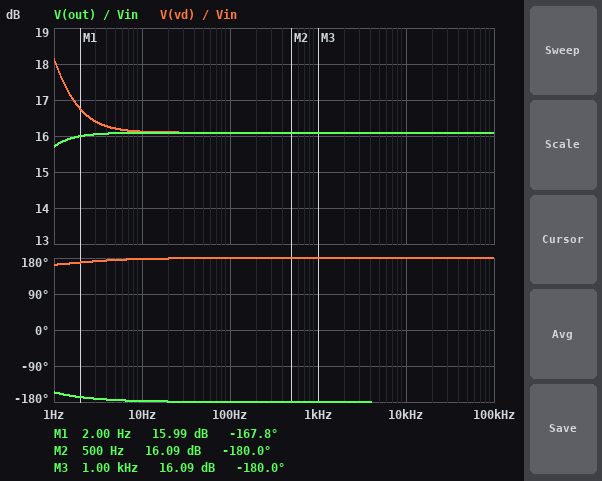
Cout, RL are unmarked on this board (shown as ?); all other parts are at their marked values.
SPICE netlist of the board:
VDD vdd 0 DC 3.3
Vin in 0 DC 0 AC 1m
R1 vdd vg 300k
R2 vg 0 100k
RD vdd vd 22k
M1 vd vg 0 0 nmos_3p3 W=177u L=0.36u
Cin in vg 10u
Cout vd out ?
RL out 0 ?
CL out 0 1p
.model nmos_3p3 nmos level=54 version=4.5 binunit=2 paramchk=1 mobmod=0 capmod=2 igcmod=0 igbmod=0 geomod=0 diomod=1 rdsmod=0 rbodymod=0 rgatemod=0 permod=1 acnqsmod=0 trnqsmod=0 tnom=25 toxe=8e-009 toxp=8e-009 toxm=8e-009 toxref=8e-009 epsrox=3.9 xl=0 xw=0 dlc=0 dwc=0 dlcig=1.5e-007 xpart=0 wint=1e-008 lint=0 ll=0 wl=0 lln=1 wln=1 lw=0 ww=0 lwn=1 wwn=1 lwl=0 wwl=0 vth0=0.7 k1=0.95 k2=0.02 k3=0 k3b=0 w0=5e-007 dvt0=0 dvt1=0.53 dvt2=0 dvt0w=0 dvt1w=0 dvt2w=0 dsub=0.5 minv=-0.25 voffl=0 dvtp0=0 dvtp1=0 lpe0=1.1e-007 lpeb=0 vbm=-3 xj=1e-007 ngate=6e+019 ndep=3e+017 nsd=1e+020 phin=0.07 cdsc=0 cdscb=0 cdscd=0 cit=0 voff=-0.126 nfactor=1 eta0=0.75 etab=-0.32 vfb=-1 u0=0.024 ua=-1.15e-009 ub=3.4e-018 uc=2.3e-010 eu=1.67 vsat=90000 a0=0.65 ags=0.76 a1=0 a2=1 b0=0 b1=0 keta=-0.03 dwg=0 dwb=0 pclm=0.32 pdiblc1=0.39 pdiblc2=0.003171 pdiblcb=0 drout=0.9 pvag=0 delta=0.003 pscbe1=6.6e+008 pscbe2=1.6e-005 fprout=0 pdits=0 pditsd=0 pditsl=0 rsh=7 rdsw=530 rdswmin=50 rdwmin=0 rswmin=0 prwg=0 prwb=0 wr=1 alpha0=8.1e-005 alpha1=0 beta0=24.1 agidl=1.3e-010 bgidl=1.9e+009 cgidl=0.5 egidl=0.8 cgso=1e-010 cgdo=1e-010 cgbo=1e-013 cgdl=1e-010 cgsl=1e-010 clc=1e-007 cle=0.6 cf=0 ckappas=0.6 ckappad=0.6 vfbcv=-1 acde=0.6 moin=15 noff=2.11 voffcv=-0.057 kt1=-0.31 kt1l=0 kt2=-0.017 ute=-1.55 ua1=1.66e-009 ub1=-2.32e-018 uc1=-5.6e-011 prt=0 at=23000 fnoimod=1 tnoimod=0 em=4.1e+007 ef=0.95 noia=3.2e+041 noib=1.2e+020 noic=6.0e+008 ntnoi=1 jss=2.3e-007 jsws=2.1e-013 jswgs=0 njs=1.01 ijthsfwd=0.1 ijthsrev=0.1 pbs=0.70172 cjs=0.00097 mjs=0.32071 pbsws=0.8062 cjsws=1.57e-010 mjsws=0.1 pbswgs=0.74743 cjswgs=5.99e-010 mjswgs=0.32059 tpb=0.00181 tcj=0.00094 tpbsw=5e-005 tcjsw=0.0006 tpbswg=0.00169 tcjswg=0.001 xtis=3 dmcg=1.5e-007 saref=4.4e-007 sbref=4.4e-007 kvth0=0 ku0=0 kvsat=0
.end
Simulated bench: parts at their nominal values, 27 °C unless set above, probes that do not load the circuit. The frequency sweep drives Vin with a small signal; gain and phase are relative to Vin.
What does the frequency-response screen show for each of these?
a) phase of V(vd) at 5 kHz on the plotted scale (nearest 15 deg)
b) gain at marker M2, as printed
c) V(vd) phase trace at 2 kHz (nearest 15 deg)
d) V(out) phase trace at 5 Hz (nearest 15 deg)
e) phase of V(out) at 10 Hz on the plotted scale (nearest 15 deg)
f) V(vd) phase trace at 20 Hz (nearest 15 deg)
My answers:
180 deg
16.09 dB
180 deg
-180 deg
-180 deg
180 deg
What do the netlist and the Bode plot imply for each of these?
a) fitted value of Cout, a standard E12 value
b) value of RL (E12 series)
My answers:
39 µF
4.7 kΩ
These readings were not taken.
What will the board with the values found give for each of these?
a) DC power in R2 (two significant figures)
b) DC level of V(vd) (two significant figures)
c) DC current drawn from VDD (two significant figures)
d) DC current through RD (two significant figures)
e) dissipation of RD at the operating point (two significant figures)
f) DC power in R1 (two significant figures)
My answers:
6.8 µW
920 mV
120 µA
110 µA
260 µW
20 µW
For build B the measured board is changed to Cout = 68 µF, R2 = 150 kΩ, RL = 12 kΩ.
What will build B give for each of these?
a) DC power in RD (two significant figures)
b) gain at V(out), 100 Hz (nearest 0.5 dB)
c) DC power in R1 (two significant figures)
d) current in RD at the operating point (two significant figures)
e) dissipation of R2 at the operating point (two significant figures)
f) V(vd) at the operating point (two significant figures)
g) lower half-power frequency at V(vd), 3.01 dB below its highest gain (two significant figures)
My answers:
490 µW
-27.5 dB
16 µW
150 µA
8.1 µW
12 mV
160 mHz
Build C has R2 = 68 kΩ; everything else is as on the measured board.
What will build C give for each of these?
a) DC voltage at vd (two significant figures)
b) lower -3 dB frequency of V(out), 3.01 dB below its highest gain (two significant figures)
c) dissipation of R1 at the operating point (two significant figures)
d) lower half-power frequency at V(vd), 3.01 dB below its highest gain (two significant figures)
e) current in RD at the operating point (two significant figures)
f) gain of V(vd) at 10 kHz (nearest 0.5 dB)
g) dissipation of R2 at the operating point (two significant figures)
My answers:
3.2 V
350 mHz
24 µW
90 mHz
2.8 µA
-11.5 dB
5.5 µW
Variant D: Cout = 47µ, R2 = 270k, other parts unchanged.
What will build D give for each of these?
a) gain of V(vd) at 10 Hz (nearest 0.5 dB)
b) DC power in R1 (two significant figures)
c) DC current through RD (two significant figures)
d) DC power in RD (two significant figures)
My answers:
-45.5 dB
10 µW
150 µA
490 µW
